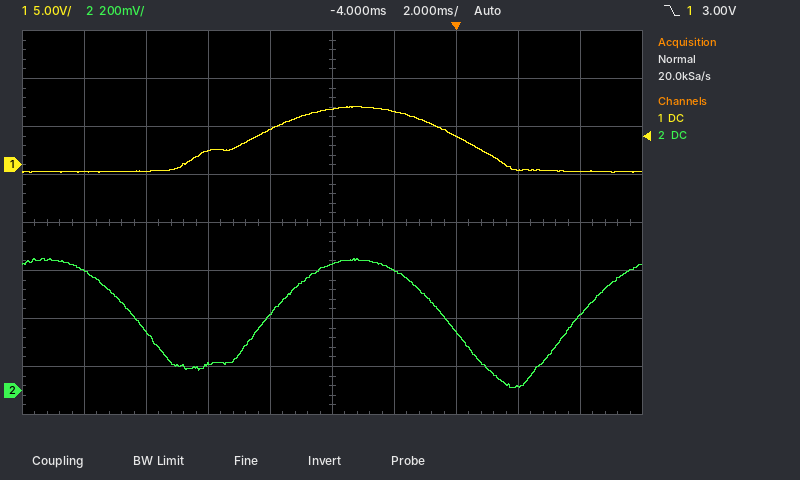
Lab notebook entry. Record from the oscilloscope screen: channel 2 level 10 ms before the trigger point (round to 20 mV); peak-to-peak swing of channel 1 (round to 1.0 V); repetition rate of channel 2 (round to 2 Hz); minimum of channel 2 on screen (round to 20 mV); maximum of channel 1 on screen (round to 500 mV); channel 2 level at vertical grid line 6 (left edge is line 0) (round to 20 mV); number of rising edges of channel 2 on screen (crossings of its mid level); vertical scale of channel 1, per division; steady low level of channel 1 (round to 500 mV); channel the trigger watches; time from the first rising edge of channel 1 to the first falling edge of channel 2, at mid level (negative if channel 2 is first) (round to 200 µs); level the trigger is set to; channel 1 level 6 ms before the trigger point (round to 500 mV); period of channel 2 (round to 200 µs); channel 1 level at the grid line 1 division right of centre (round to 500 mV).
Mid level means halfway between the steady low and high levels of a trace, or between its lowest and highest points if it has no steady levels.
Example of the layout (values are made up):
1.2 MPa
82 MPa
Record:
240 mV
7.0 V
100 Hz
20 mV
6.0 V
500 mV
2
5 V
-500 mV
channel 1
-3.6 ms
3.00 V
3.5 V
10.0 ms
5.5 V
